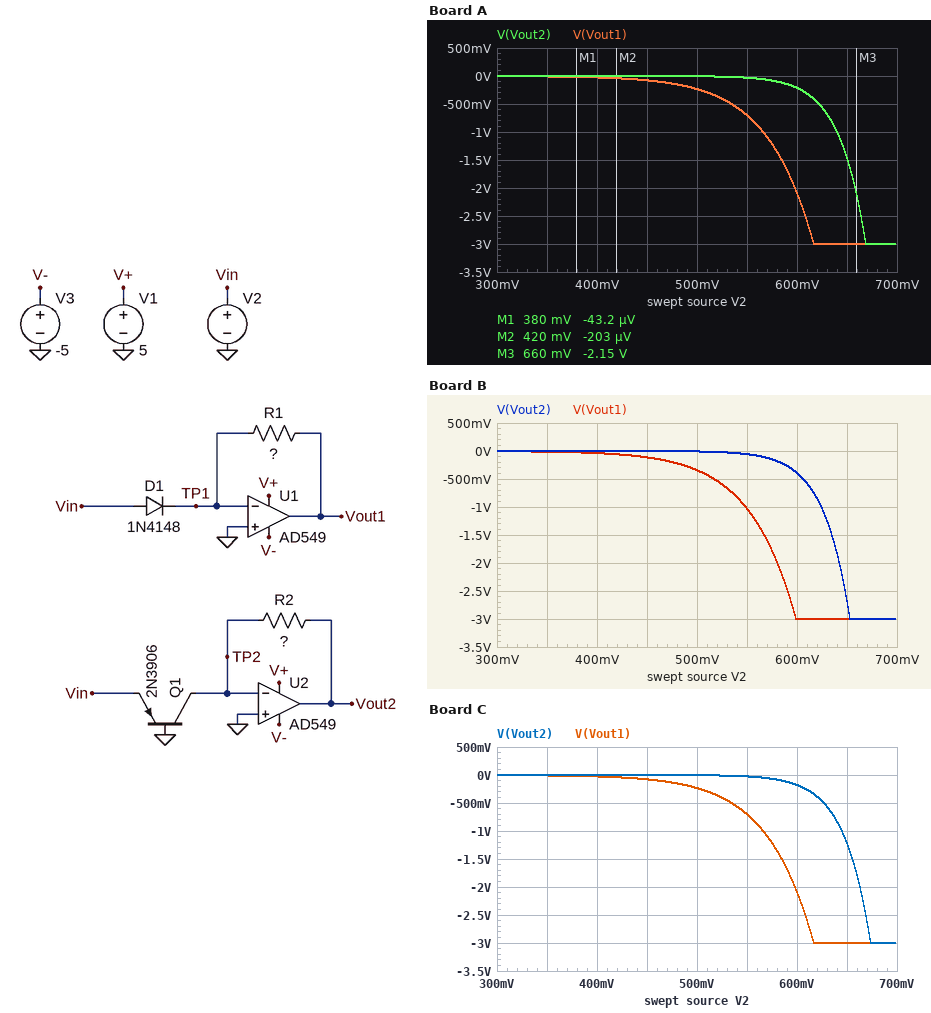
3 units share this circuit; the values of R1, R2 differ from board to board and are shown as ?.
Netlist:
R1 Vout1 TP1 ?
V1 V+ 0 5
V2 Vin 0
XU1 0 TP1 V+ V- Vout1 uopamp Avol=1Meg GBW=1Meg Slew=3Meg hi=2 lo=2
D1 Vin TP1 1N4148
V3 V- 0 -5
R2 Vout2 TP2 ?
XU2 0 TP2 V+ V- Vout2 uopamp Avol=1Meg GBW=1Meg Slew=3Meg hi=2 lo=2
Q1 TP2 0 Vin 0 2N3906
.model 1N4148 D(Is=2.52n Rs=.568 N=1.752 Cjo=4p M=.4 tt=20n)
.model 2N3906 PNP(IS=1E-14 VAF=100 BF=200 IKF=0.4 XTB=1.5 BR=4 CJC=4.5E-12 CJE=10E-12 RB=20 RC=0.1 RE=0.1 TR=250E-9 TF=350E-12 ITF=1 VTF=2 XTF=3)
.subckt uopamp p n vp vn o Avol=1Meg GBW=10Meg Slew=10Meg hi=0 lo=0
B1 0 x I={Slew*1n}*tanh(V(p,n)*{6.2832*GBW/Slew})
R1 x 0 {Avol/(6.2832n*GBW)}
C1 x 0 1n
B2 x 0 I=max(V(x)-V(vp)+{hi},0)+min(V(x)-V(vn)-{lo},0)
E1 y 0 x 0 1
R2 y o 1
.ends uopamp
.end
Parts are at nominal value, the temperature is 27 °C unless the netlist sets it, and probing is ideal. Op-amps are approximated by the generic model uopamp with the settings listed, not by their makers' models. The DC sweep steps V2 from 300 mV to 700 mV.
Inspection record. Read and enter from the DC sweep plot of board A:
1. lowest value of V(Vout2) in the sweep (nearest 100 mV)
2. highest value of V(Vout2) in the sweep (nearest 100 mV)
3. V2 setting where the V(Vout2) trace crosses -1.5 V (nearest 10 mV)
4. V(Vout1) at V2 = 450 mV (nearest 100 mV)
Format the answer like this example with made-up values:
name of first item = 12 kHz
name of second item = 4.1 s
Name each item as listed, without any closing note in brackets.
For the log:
lowest value of V(Vout2) in the sweep = -3.0 V
highest value of V(Vout2) in the sweep = 0 V
V2 setting where the V(Vout2) trace crosses -1.5 V = 650 mV
V(Vout1) at V2 = 450 mV = -100 mV
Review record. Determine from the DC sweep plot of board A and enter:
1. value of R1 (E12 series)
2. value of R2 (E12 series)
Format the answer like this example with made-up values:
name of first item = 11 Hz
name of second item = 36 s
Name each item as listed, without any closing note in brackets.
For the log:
value of R1 = 1.5 kΩ
value of R2 = 1.8 kΩ
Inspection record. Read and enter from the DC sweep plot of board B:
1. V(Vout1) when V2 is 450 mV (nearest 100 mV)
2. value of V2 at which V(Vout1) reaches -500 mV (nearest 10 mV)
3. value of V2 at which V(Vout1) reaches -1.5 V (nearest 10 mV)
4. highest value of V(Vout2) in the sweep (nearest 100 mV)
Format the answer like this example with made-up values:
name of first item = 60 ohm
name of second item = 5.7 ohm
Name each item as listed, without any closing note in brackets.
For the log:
V(Vout1) when V2 is 450 mV = -100 mV
value of V2 at which V(Vout1) reaches -500 mV = 520 mV
value of V2 at which V(Vout1) reaches -1.5 V = 570 mV
highest value of V(Vout2) in the sweep = 0 V
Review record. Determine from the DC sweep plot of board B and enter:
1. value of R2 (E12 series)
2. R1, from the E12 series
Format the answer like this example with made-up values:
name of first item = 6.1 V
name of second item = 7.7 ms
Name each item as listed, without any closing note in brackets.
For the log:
value of R2 = 3.3 kΩ
R1, from the E12 series = 2.2 kΩ
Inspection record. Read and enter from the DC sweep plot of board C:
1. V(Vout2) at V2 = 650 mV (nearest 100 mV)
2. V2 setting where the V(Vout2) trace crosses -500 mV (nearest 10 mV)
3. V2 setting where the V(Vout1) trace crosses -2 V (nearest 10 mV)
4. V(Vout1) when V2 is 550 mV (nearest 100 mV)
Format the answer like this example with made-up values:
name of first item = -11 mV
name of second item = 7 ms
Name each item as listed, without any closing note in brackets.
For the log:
V(Vout2) at V2 = 650 mV = -1.2 V
V2 setting where the V(Vout2) trace crosses -500 mV = 630 mV
V2 setting where the V(Vout1) trace crosses -2 V = 600 mV
V(Vout1) when V2 is 550 mV = -700 mV
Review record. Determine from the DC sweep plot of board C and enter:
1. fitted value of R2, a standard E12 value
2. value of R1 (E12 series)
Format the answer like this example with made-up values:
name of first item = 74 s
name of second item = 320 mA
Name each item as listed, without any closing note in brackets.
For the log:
fitted value of R2, a standard E12 value = 1.5 kΩ
value of R1 = 1.5 kΩ
